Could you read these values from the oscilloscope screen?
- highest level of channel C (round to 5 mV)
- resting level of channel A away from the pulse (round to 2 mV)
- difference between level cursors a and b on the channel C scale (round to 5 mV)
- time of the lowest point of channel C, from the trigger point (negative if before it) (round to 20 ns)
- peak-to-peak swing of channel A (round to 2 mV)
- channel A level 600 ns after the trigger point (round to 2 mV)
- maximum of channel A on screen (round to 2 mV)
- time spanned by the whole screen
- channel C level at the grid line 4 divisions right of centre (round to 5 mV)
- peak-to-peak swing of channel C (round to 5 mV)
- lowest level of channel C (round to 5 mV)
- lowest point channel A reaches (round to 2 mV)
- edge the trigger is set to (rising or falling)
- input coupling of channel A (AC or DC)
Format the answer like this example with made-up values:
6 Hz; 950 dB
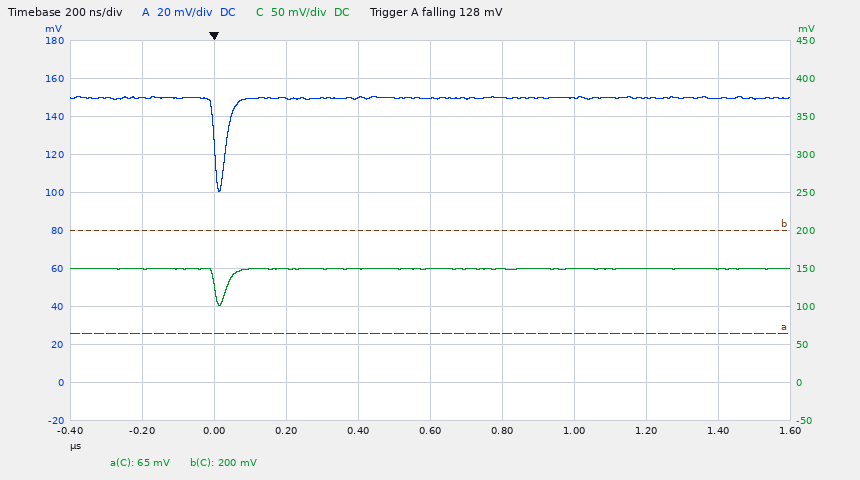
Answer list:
150 mV; 150 mV; 135 mV; +20 ns; 50 mV; 150 mV; 150 mV; 2 µs; 150 mV; 50 mV; 100 mV; 100 mV; falling; DC
